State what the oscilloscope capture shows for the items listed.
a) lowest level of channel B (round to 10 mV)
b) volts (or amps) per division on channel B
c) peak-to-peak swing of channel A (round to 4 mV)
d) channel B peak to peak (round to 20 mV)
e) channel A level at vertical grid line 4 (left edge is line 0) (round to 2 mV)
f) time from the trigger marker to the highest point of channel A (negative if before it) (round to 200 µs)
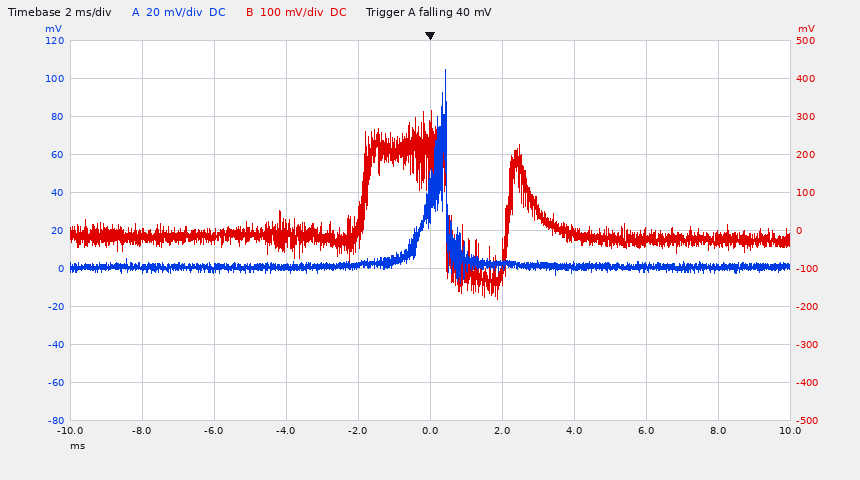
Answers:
-180 mV
100 mV
112 mV
500 mV
2 mV
+400 µs
